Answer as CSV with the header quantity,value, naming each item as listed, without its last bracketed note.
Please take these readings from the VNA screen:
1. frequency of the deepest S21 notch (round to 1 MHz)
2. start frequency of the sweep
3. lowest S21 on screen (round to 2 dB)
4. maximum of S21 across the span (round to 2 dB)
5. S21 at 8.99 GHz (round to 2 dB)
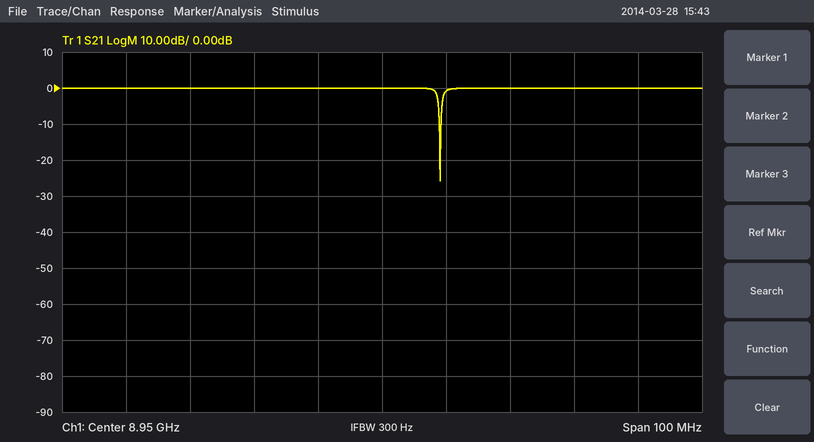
quantity,value
frequency of the deepest S21 notch,8.959 GHz
start frequency of the sweep,8.9 GHz
lowest S21 on screen,-26 dB
maximum of S21 across the span,0 dB
S21 at 8.99 GHz,0 dB
